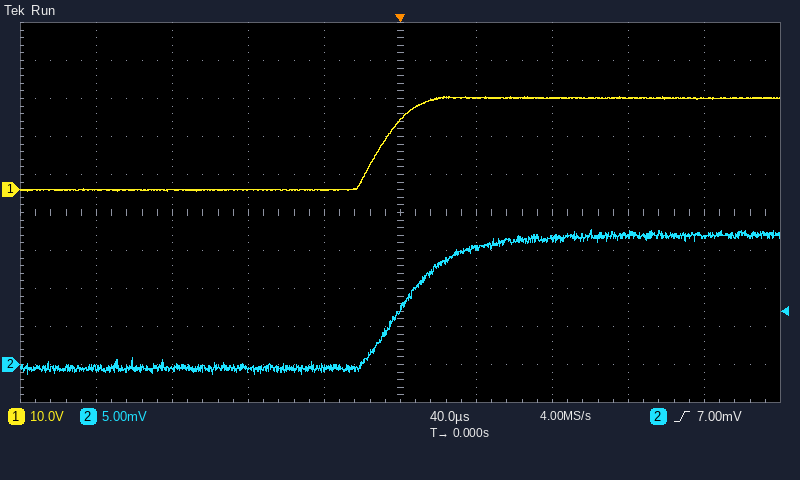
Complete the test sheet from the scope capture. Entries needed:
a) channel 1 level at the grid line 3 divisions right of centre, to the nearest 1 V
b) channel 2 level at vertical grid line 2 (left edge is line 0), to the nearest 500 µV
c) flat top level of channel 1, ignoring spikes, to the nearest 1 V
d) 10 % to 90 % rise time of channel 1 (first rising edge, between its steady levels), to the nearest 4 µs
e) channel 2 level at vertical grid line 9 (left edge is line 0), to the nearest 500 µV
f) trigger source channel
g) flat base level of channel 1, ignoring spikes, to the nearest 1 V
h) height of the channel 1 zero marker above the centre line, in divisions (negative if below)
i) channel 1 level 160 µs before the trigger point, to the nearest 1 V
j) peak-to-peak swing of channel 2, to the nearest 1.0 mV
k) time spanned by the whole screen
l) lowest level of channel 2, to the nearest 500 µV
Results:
24 V
-500 µV
24 V
28 µs
17.0 mV
channel 2
0 V
+0.6 div
0 V
19.0 mV
400 µs
-1.5 mV
